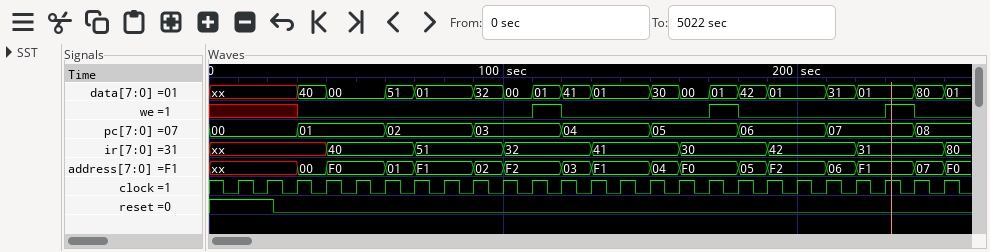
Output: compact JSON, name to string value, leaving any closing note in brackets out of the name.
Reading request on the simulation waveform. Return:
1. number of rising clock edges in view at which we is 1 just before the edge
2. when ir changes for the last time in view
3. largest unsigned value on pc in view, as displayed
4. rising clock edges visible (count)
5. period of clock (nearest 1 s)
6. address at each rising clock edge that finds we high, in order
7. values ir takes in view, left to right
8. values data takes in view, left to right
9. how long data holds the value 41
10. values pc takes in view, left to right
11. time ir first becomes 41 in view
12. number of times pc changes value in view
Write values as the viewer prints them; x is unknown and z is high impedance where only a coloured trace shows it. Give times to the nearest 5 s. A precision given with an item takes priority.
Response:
{"number of rising clock edges in view at which we is 1 just before the edge": "3", "when ir changes for the last time in view": "250 s", "largest unsigned value on pc in view, as displayed": "08", "rising clock edges visible": "25", "period of clock": "10 s", "address at each rising clock edge that finds we high, in order": "F2, F0, F1", "values ir takes in view, left to right": "xx, 40, 51, 32, 41, 30, 42, 31, 80", "values data takes in view, left to right": "xx, 40, 00, 51, 01, 32, 00, 01, 41, 01, 30, 00, 01, 42, 01, 31, 01, 80, 01", "how long data holds the value 41": "10 s", "values pc takes in view, left to right": "00, 01, 02, 03, 04, 05, 06, 07, 08", "time ir first becomes 41 in view": "130 s", "number of times pc changes value in view": "8"}
